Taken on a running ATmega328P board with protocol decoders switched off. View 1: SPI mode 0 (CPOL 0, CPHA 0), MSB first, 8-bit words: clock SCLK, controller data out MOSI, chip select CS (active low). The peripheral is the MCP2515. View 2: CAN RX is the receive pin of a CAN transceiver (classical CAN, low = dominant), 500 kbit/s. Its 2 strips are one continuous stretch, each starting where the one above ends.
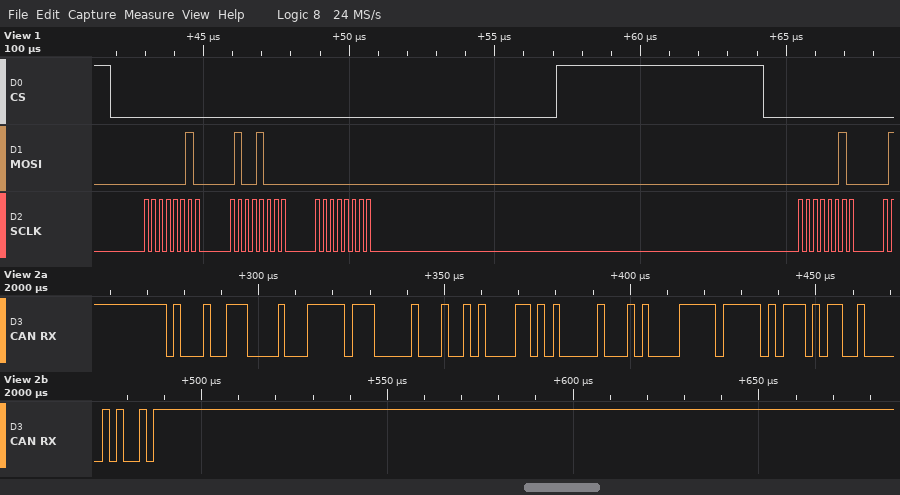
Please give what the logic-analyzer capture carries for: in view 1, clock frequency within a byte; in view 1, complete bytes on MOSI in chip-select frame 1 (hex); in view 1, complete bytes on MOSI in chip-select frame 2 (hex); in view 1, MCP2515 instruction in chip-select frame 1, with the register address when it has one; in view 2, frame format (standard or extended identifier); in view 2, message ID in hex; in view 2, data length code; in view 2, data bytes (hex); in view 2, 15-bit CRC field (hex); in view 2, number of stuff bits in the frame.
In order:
4 MHz
02 48 00
02
WRITE 0x48
standard
0x44E
8
FF 00 94 35 00 A1 FF DD
0x3204
6
